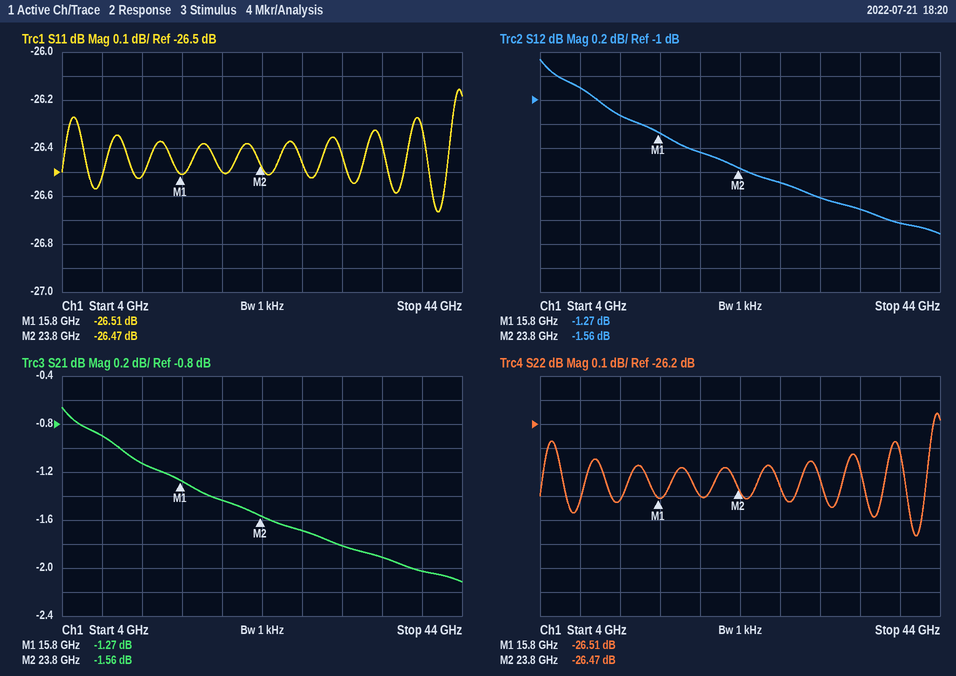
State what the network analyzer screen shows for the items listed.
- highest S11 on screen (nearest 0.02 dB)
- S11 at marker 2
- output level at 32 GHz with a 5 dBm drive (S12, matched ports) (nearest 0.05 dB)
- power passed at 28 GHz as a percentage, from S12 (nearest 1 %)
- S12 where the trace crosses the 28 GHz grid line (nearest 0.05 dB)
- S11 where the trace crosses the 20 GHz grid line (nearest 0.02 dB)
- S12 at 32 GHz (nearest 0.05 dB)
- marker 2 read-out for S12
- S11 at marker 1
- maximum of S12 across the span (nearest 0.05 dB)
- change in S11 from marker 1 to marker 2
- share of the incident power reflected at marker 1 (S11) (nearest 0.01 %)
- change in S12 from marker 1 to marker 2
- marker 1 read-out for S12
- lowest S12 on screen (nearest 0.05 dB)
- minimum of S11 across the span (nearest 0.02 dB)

-26.16 dB
-26.47 dB
3.20 dBm
68 %
-1.70 dB
-26.50 dB
-1.80 dB
-1.56 dB
-26.51 dB
-0.65 dB
0.04 dB
0.22 %
-0.29 dB
-1.27 dB
-2.10 dB
-26.66 dB
